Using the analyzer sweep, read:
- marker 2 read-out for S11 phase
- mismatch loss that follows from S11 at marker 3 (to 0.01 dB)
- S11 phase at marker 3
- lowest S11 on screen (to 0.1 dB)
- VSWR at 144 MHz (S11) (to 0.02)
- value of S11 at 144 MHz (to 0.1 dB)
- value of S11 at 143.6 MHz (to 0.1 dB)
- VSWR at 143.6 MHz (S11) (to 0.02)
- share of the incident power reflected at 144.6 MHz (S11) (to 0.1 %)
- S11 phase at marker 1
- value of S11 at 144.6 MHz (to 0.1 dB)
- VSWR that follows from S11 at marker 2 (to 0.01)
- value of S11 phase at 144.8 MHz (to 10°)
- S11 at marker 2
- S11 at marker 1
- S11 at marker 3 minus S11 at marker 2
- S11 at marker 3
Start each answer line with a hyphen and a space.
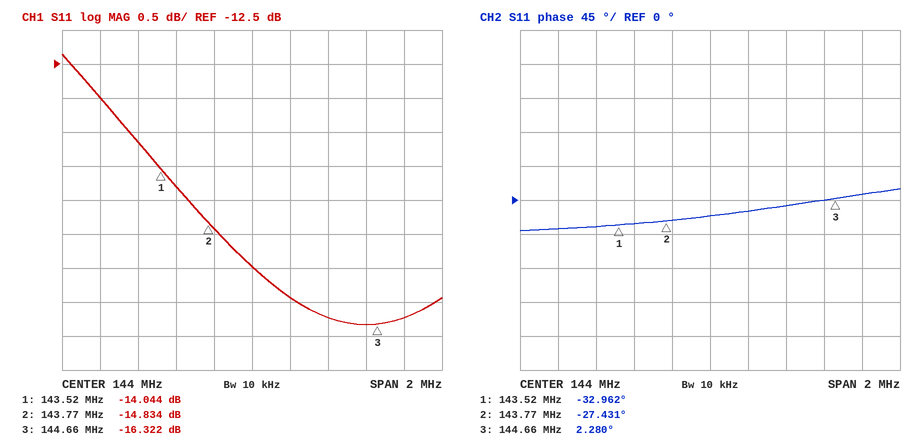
- -27.431°
- 0.10 dB
- 2.280°
- -16.3 dB
- 1.40
- -15.5 dB
- -14.3 dB
- 1.48
- 2.3 %
- -32.962°
- -16.3 dB
- 1.44
- 10°
- -14.834 dB
- -14.044 dB
- -1.488 dB
- -16.322 dB
